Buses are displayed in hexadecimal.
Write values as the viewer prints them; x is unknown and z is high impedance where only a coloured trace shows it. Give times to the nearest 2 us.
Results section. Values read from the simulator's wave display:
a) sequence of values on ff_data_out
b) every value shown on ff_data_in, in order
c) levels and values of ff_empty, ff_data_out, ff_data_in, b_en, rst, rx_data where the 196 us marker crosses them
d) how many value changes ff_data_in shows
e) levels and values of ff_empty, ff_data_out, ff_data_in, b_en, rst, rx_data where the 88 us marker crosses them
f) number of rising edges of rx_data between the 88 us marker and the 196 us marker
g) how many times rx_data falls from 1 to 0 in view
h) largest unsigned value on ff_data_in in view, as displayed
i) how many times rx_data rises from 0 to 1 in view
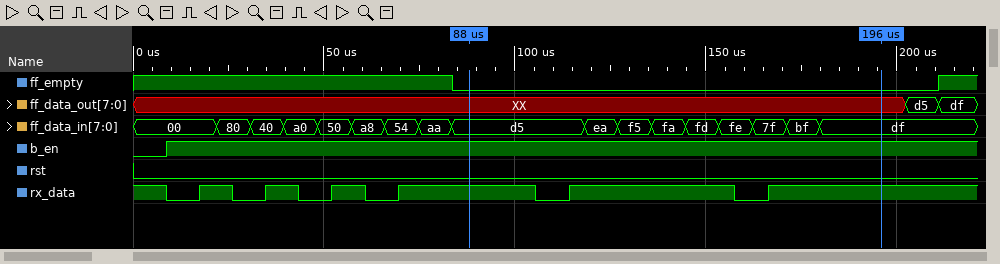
XX, d5, df
00, 80, 40, a0, 50, a8, 54, aa, d5, ea, f5, fa, fd, fe, 7f, bf, df
ff_empty=0, ff_data_out=XX, ff_data_in=df, b_en=1, rst=0, rx_data=1
16
ff_empty=0, ff_data_out=XX, ff_data_in=d5, b_en=1, rst=0, rx_data=1
2
6
fe
6
